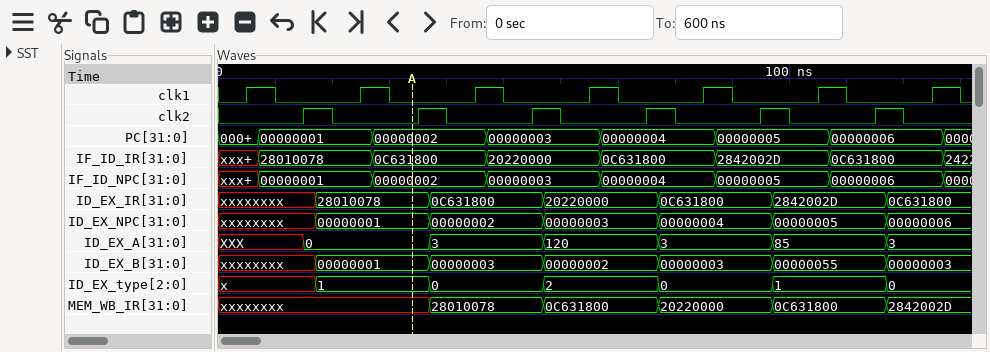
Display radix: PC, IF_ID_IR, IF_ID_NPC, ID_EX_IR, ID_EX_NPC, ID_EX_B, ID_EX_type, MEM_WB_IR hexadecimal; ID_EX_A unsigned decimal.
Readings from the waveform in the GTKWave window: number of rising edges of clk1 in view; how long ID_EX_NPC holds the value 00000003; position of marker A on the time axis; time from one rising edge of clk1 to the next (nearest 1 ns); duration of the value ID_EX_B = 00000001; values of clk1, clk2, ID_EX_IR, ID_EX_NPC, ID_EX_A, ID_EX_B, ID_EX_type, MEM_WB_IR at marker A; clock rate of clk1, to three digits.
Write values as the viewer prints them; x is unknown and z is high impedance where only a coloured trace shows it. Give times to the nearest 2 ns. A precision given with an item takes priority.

7
20 ns
34 ns
20 ns
20 ns
clk1=0, clk2=0, ID_EX_IR=28010078, ID_EX_NPC=00000001, ID_EX_A=0, ID_EX_B=00000001, ID_EX_type=1, MEM_WB_IR=xxxxxxxx
50.0 MHz
